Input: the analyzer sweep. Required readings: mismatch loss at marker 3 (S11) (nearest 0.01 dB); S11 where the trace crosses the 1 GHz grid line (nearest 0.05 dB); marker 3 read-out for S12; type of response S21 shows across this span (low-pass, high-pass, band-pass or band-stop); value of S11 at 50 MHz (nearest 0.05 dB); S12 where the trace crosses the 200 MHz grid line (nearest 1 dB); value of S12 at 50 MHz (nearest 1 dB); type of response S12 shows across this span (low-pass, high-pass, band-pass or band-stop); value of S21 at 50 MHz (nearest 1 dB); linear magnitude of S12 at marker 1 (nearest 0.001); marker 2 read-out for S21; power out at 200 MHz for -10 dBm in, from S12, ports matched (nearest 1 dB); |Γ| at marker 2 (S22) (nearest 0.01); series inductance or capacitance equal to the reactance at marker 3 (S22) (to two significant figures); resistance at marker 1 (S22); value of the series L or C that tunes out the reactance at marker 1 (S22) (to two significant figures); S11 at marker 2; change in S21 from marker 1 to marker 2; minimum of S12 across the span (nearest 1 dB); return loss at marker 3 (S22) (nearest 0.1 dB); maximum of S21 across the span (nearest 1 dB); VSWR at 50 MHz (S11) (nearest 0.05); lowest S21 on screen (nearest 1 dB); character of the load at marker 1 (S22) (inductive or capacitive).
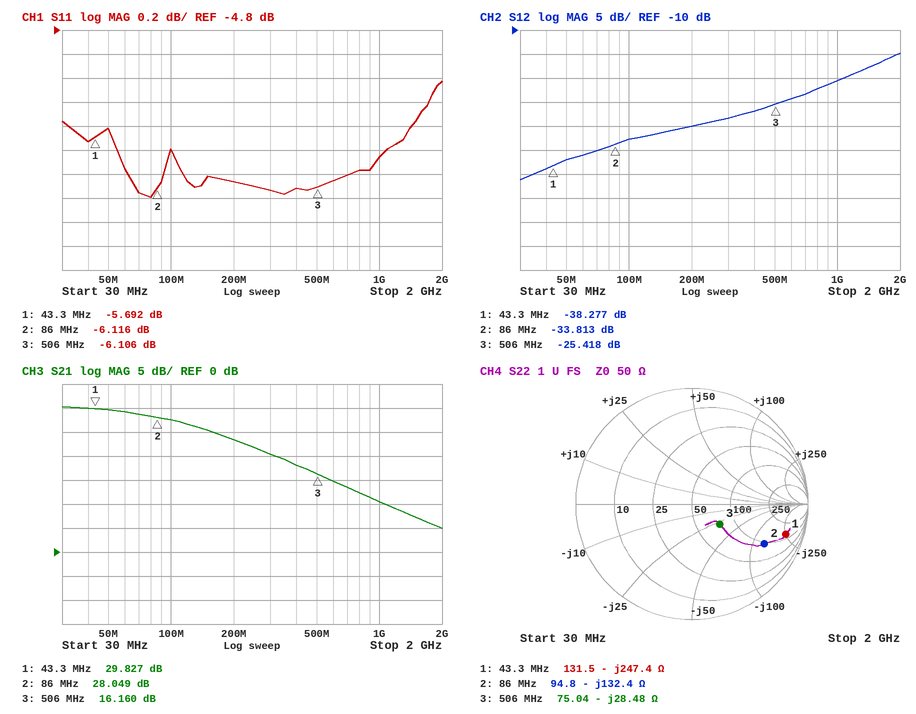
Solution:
1.22 dB
-5.85 dB
-25.418 dB
low-pass
-5.60 dB
-30 dB
-37 dB
high-pass
30 dB
0.012
28.049 dB
-40 dBm
0.71
11 pF
131.5 Ω
910 nH
-6.116 dB
-1.778 dB
-41 dB
10.6 dB
30 dB
3.20
5 dB
capacitive
